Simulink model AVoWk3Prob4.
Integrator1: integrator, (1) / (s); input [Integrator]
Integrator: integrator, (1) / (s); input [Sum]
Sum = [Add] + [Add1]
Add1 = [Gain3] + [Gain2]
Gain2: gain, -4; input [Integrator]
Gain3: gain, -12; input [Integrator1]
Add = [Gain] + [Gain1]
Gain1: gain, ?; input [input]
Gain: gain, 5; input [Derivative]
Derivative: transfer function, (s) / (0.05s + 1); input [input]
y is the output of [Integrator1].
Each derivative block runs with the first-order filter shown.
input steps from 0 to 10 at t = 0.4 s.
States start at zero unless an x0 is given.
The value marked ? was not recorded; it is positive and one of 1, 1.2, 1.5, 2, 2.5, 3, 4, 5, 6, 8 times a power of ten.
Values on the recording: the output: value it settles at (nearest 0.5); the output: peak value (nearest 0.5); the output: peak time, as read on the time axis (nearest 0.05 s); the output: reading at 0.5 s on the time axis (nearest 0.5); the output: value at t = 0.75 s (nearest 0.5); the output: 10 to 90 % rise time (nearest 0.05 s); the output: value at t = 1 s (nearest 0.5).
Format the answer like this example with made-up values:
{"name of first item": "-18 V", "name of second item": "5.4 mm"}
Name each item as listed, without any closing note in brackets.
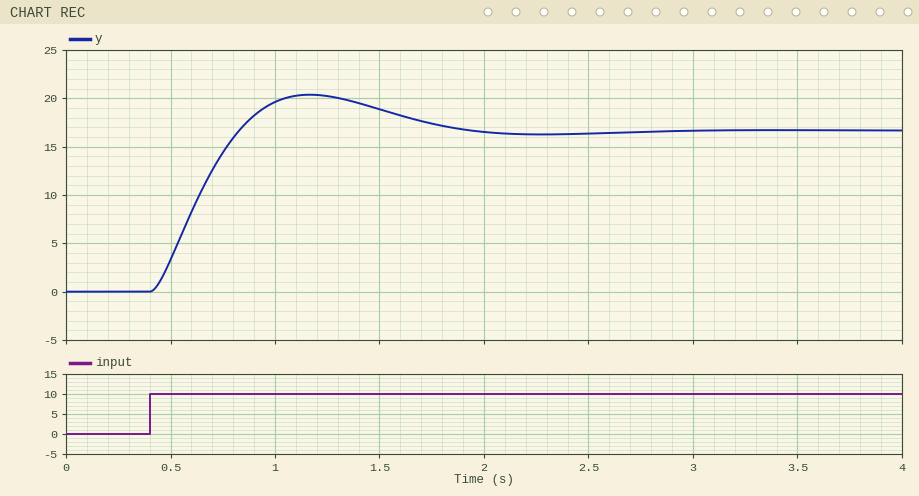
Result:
{"the output: value it settles at": "16.5", "the output: peak value": "20.5", "the output: peak time, as read on the time axis": "1.15 s", "the output: reading at 0.5 s on the time axis": "3.5", "the output: value at t = 0.75 s": "14.5", "the output: 10 to 90 % rise time": "0.30 s", "the output: value at t = 1 s": "19.5"}
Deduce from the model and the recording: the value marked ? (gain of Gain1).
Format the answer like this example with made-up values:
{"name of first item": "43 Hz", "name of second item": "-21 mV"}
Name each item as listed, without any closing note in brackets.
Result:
{"the value marked ?": "20"}
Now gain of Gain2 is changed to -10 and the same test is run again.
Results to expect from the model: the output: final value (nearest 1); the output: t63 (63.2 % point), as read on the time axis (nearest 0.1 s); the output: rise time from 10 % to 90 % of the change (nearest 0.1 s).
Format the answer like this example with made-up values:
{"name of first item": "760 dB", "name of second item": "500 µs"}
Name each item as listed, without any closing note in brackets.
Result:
{"the output: final value": "17", "the output: t63 (63.2 % point), as read on the time axis": "0.9 s", "the output: rise time from 10 % to 90 % of the change": "1.4 s"}
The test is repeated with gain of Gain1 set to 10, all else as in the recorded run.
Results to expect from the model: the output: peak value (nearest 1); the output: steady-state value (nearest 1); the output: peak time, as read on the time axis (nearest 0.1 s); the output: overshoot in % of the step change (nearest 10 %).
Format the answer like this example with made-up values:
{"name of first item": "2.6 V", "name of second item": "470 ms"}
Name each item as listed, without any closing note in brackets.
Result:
{"the output: peak value": "13", "the output: steady-state value": "8", "the output: peak time, as read on the time axis": "1.0 s", "the output: overshoot in % of the step change": "50 %"}
